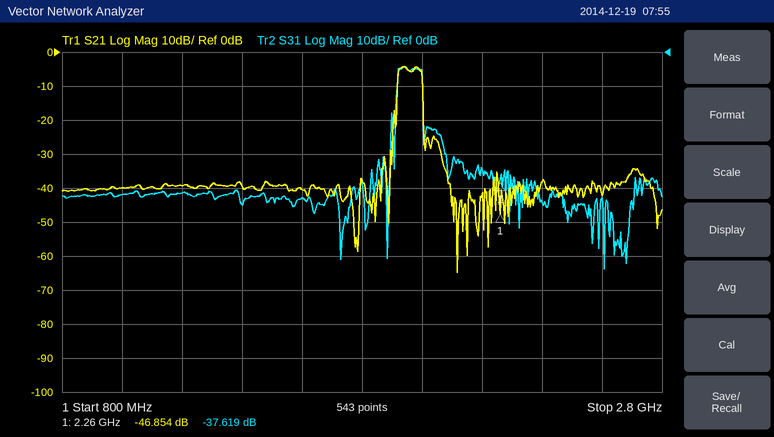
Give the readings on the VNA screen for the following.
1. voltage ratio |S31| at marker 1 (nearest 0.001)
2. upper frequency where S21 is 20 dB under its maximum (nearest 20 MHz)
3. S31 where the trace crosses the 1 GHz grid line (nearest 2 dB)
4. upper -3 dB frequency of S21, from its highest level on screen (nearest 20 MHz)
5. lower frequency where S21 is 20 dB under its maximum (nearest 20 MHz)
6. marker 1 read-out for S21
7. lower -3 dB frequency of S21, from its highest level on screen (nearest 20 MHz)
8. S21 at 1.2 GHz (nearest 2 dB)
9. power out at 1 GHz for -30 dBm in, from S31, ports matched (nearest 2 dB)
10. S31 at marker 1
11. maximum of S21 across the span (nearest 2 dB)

0.013
2.00 GHz
-42 dB
2.00 GHz
1.90 GHz
-46.854 dB
1.92 GHz
-40 dB
-72 dBm
-37.619 dB
-4 dB
